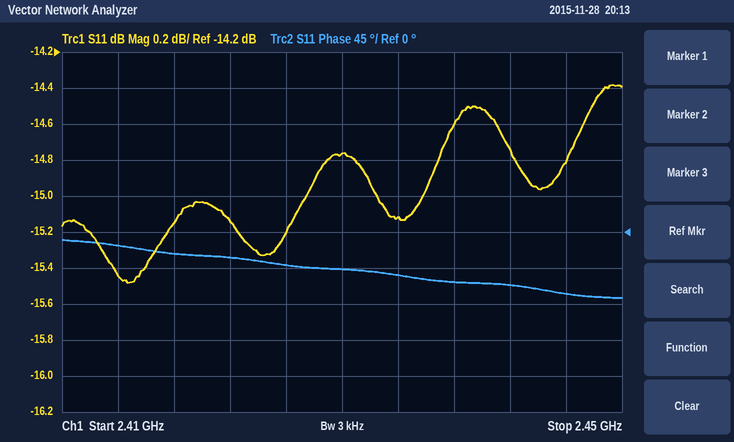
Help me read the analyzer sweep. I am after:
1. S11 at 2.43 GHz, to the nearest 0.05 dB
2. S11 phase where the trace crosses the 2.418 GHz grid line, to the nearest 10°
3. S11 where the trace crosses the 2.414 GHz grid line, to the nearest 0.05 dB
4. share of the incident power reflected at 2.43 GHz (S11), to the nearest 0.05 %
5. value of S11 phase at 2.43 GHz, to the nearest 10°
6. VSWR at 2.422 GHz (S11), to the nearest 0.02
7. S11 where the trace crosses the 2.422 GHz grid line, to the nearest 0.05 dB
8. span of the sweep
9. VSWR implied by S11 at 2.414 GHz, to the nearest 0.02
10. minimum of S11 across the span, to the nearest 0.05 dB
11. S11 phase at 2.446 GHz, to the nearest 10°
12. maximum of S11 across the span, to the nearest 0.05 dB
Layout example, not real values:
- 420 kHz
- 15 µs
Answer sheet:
- -14.75 dB
- -30°
- -15.45 dB
- 3.35 %
- -50°
- 1.42
- -15.15 dB
- 40 MHz
- 1.40
- -15.50 dB
- -80°
- -14.40 dB
